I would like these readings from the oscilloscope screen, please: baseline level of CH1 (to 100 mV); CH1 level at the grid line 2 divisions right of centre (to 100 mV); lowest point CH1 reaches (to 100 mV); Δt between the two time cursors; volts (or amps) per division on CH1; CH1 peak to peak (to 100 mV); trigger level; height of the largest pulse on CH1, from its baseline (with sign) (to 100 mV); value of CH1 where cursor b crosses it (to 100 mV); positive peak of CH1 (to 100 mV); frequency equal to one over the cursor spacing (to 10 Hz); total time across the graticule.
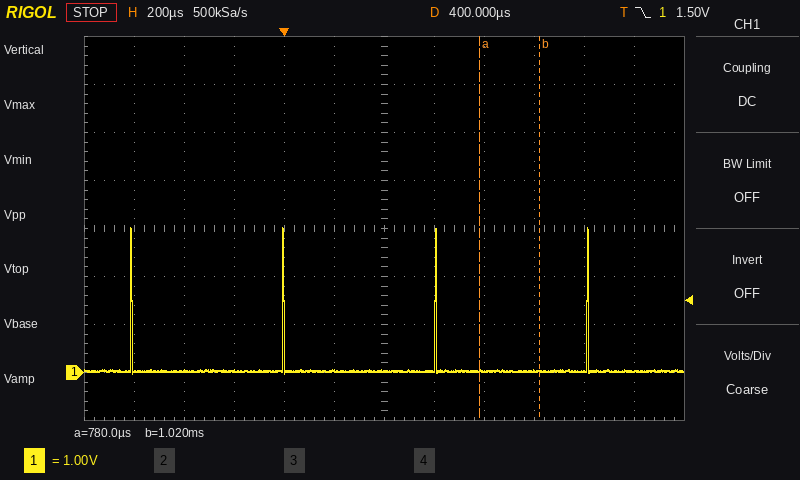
0.0 V
0.0 V
0.0 V
240 µs
1 V
3.0 V
1.50 V
+3.0 V
0.0 V
3.0 V
4.17 kHz
2.4 ms
